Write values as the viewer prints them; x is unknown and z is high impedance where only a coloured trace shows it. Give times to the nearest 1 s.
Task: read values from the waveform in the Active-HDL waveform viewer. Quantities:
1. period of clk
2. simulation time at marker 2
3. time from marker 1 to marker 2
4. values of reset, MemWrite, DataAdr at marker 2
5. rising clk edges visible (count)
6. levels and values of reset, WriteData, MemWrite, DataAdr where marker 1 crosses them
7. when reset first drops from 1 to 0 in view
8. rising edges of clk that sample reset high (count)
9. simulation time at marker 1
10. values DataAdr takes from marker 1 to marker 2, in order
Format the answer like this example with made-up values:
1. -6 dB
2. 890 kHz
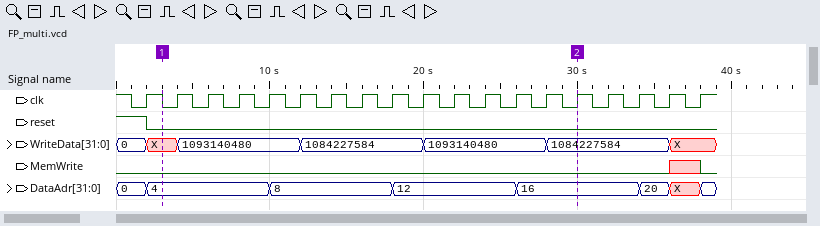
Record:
1. 2 s
2. 30 s
3. 27 s
4. reset=0, MemWrite=0, DataAdr=16
5. 19
6. reset=0, WriteData=X, MemWrite=0, DataAdr=4
7. 2 s
8. 1
9. 3 s
10. 4, 8, 12, 16
